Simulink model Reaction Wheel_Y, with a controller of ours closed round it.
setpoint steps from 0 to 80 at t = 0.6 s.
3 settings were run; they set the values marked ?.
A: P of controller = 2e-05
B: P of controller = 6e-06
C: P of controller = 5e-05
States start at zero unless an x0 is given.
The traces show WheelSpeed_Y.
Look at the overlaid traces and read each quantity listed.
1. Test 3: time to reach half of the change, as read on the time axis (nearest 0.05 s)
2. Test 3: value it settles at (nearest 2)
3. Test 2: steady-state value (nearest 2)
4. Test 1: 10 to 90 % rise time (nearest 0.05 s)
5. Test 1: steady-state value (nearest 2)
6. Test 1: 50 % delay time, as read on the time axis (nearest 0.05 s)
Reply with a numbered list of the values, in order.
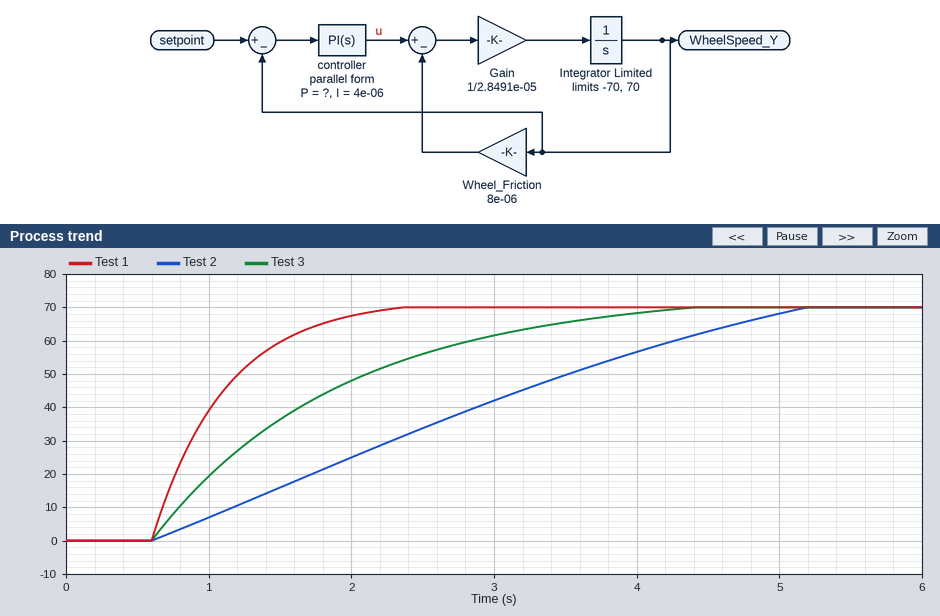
1. 1.45 s
2. 70
3. 70
4. 1.00 s
5. 70
6. 0.95 s
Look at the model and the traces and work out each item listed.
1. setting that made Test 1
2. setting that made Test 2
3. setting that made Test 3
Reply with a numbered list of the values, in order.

1. C
2. B
3. A
